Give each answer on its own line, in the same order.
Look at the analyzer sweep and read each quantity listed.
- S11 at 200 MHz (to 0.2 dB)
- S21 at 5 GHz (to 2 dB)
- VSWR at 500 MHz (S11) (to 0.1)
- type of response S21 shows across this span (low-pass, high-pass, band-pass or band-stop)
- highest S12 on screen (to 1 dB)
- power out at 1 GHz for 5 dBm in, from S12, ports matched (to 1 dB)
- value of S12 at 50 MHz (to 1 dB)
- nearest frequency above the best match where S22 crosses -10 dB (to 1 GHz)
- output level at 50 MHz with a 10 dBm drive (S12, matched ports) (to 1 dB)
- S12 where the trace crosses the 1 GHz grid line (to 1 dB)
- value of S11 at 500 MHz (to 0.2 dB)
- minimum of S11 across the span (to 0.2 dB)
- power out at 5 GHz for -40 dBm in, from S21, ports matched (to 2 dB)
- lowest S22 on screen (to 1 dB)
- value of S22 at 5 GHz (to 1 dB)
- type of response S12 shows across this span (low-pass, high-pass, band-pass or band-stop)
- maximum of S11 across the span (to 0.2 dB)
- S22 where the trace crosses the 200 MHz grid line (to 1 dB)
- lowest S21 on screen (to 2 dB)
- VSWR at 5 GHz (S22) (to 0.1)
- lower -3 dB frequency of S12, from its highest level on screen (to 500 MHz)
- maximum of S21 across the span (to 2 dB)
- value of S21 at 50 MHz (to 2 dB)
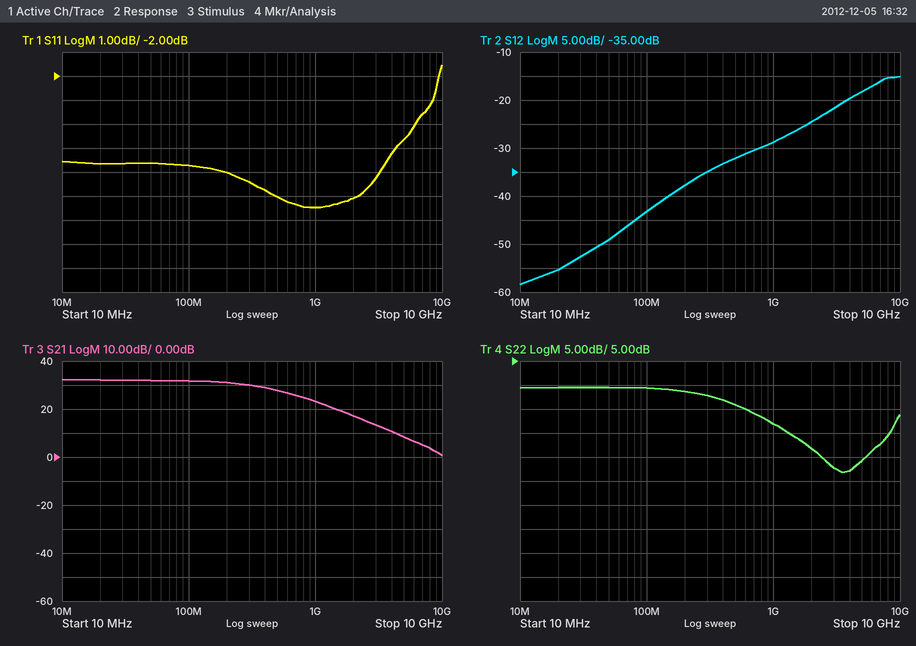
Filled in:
-6.0 dB
8 dB
2.6
low-pass
-15 dB
-24 dBm
-49 dB
8 GHz
-39 dBm
-29 dB
-7.0 dB
-7.4 dB
-32 dBm
-18 dB
-16 dB
high-pass
-1.6 dB
-1 dB
0 dB
1.4
5.0 GHz
32 dB
32 dB
